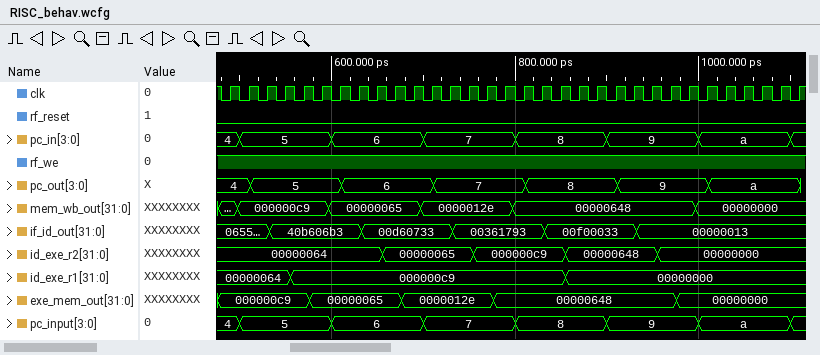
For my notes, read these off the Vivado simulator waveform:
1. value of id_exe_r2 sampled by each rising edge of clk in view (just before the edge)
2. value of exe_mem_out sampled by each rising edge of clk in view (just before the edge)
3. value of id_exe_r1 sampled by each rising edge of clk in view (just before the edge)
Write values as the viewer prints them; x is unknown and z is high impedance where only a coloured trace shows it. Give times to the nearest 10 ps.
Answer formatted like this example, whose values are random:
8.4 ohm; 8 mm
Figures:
00000064, 00000064, 00000064, 00000064, 00000064, 00000064, 00000064, 00000064, 00000064, 00000065, 00000065, 00000065, 00000065, 00000065, 000000c9, 000000c9, 000000c9, 000000c9, 000000c9, 00000648, 00000648, 00000648, 00000648, 00000648, 00000000, 00000000, 00000000, 00000000, 00000000, 00000000, 00000000, 00000000; 000000c9, 000000c9, 000000c9, 000000c9, 000000c9, 00000065, 00000065, 00000065, 00000065, 00000065, 0000012e, 0000012e, 0000012e, 0000012e, 0000012e, 00000648, 00000648, 00000648, 00000648, 00000648, 00000648, 00000648, 00000648, 00000648, 00000648, 00000000, 00000000, 00000000, 00000000, 00000000, 00000000, 00000000; 00000064, 00000064, 00000064, 00000064, 000000c9, 000000c9, 000000c9, 000000c9, 000000c9, 000000c9, 000000c9, 000000c9, 000000c9, 000000c9, 000000c9, 000000c9, 000000c9, 000000c9, 000000c9, 00000000, 00000000, 00000000, 00000000, 00000000, 00000000, 00000000, 00000000, 00000000, 00000000, 00000000, 00000000, 00000000
